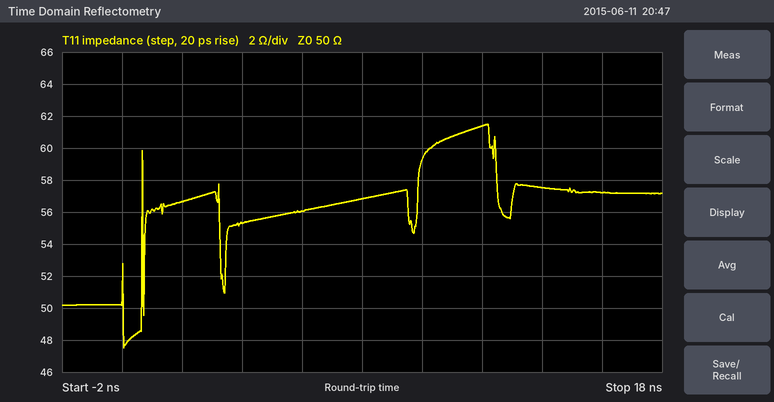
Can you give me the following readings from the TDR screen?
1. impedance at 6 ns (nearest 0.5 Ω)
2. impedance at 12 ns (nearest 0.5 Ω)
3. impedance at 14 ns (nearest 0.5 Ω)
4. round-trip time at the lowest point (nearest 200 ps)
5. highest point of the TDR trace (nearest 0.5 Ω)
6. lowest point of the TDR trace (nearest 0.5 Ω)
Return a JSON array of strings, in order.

["56.0 Ω", "61.5 Ω", "57.5 Ω", "0.0 ns", "61.5 Ω", "47.5 Ω"]
